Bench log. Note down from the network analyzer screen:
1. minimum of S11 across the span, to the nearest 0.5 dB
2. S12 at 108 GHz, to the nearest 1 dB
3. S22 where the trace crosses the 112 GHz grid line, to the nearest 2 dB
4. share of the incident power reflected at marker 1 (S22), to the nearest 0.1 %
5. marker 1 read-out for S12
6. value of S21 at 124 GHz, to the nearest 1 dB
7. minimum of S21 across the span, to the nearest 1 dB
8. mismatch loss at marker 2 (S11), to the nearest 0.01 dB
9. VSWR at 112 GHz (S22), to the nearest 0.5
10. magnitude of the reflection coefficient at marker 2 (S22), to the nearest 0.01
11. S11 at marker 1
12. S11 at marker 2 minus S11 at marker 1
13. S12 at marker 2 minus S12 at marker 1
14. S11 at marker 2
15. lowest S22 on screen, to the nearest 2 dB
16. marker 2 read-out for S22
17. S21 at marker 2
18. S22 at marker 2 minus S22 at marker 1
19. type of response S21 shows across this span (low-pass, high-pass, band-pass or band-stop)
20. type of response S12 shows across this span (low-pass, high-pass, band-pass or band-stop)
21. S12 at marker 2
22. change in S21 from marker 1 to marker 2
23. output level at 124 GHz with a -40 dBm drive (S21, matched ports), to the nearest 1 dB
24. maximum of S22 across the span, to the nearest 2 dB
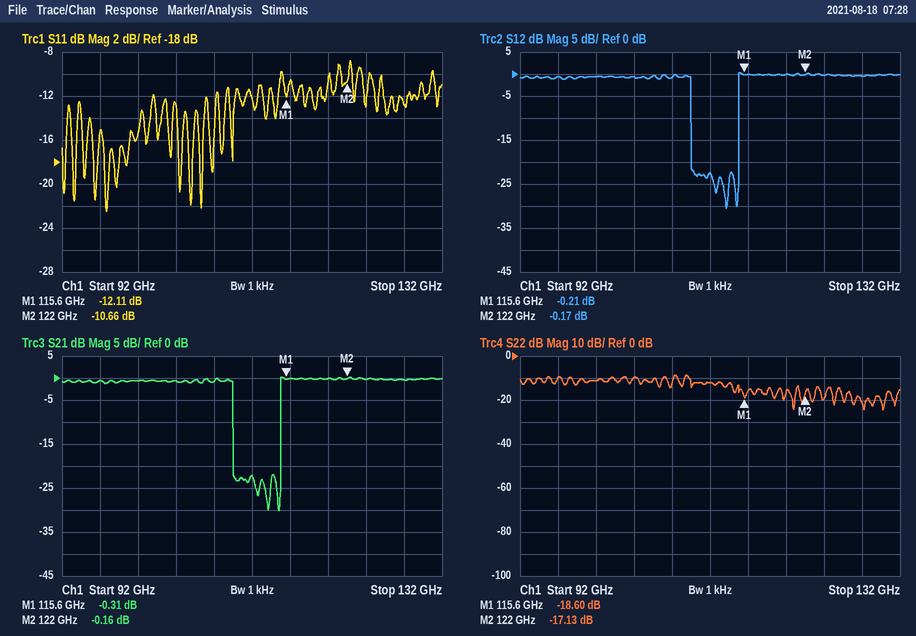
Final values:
-22.5 dB
-1 dB
-12 dB
1.4 %
-0.21 dB
0 dB
-30 dB
0.39 dB
1.5
0.14
-12.11 dB
1.45 dB
0.04 dB
-10.66 dB
-24 dB
-17.13 dB
-0.16 dB
1.47 dB
band-stop
band-stop
-0.17 dB
0.15 dB
-40 dBm
-8 dB
